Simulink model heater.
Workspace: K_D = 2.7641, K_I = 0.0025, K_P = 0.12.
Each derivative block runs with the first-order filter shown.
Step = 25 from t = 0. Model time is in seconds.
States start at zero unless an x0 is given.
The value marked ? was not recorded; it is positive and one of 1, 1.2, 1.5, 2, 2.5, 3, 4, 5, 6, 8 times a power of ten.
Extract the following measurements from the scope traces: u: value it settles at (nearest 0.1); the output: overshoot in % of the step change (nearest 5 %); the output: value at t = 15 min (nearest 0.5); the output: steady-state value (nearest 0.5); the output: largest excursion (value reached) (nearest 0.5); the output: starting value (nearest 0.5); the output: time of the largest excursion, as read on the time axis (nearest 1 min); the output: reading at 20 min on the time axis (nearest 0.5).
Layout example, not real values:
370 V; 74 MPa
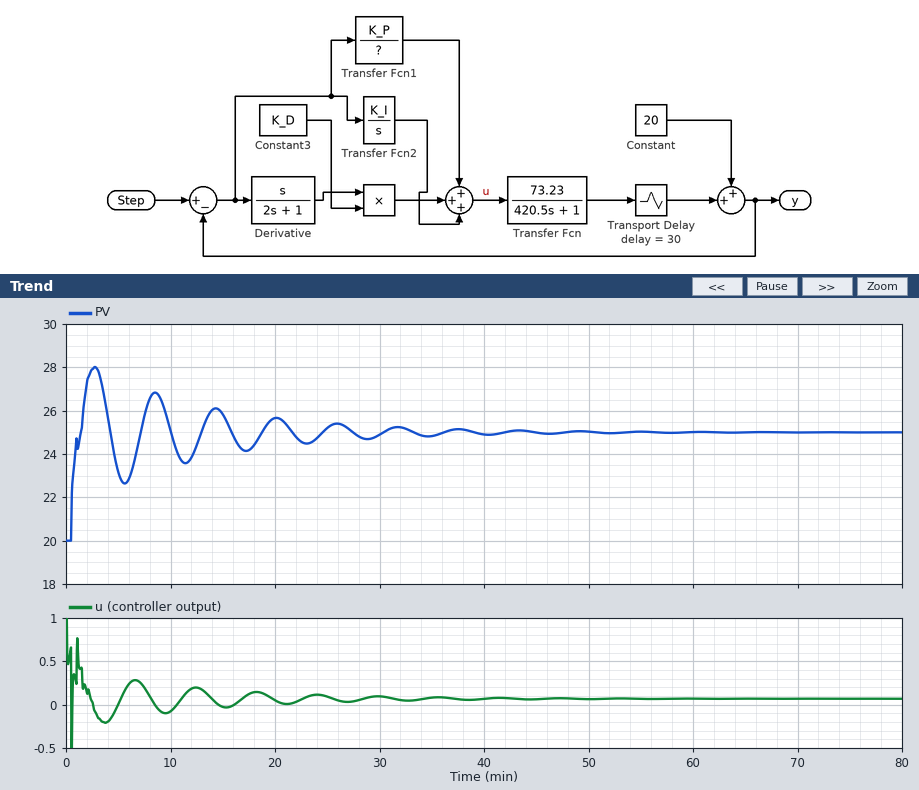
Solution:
0.1; 60 %; 26.0; 25.0; 28.0; 20.0; 3 min; 25.5
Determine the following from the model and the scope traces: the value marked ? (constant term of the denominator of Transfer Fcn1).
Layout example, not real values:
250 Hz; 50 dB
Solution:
2
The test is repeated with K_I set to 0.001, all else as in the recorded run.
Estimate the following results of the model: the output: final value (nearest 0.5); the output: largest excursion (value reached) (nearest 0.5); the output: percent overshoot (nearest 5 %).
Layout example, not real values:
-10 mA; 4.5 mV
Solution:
25.0; 26.5; 30 %
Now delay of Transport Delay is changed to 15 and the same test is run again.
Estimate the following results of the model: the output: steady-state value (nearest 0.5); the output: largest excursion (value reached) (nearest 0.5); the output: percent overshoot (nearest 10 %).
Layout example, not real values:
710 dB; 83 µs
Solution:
25.0; 27.0; 40 %
